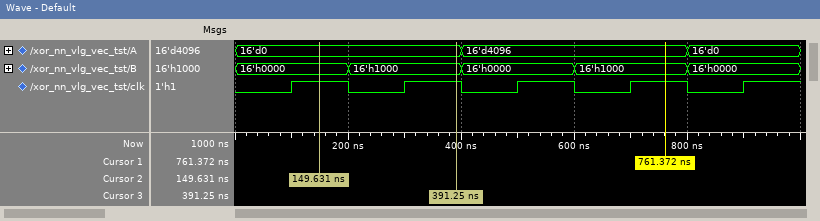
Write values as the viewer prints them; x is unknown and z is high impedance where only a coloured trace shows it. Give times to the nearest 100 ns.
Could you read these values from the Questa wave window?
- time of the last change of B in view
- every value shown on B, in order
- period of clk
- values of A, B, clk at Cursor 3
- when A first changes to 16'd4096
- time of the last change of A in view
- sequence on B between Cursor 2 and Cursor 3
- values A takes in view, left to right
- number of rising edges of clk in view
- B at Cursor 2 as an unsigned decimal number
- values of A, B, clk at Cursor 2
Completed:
800 ns
16'h0000, 16'h1000, 16'h0000, 16'h1000, 16'h0000
200 ns
A=16'd0, B=16'h1000, clk=1
400 ns
800 ns
16'h0000, 16'h1000
16'd0, 16'd4096, 16'd0
5
0
A=16'd0, B=16'h0000, clk=1
